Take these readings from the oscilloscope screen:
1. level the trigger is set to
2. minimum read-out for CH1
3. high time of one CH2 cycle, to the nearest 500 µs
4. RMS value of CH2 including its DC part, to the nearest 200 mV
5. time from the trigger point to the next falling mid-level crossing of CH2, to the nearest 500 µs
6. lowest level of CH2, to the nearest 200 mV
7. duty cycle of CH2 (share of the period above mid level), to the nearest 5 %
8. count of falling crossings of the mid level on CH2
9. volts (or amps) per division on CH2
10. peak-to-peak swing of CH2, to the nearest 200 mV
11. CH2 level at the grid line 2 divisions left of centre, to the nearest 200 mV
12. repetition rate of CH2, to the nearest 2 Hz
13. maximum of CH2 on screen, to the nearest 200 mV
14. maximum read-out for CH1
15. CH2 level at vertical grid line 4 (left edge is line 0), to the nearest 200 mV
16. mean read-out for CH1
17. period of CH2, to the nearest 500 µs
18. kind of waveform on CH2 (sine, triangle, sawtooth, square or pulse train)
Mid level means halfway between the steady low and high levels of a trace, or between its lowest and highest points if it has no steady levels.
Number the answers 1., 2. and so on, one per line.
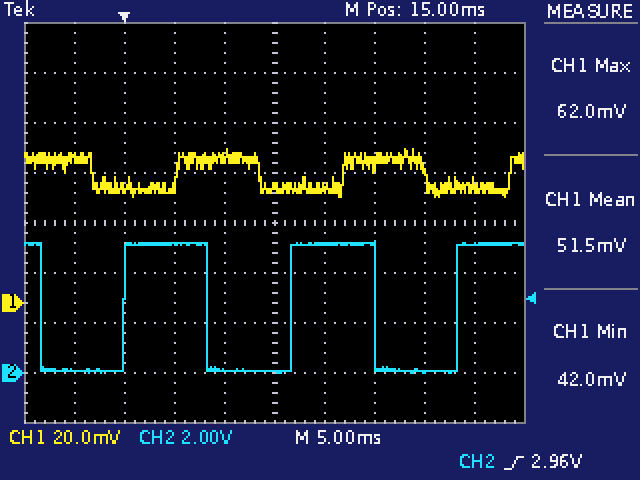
1. 2.96 V
2. 42.0 mV
3. 8.5 ms
4. 3.6 V
5. 8.5 ms
6. 0.0 V
7. 50 %
8. 3
9. 2 V
10. 5.2 V
11. 5.2 V
12. 60 Hz
13. 5.2 V
14. 62.0 mV
15. 200 mV
16. 51.5 mV
17. 16.5 ms
18. square
